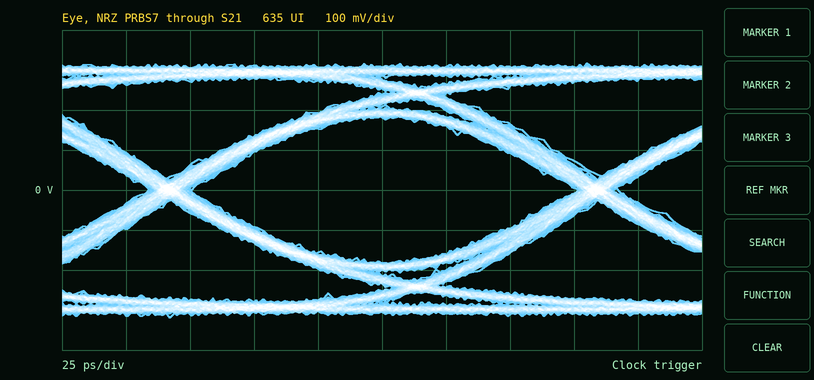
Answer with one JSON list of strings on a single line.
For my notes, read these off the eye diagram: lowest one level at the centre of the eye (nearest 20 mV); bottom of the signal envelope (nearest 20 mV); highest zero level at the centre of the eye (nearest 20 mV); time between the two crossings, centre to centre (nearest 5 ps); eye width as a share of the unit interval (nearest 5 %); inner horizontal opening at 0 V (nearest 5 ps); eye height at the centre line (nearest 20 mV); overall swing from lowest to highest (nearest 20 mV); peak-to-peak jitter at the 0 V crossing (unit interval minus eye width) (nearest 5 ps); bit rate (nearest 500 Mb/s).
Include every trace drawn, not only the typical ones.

["180 mV", "-320 mV", "-180 mV", "165 ps", "90 %", "150 ps", "360 mV", "640 mV", "15 ps", "6.0 Gb/s"]
